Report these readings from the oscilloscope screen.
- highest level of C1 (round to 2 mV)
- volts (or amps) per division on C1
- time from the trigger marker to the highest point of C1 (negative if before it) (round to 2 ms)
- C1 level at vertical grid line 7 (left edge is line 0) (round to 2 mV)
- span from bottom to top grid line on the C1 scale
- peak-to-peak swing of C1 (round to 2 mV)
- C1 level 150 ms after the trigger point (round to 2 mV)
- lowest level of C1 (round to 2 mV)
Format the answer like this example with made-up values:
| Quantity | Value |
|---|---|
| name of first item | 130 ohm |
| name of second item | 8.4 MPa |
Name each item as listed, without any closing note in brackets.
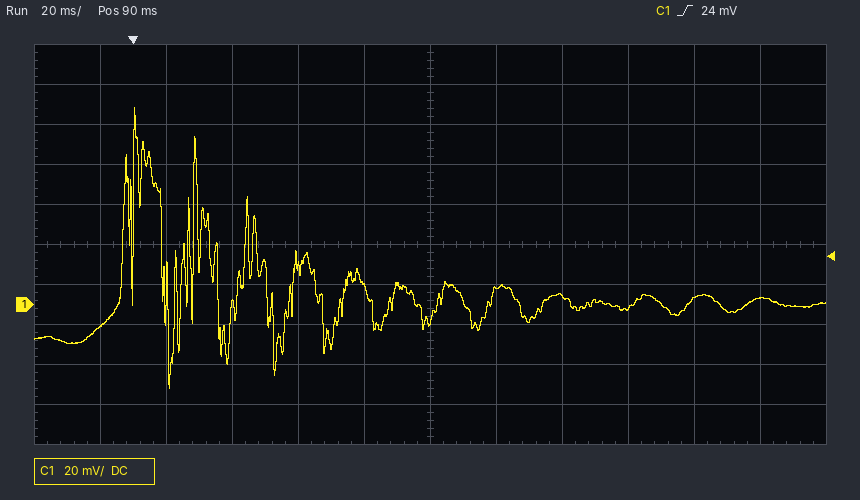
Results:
| Quantity | Value |
|---|---|
| highest level of C1 | 98 mV |
| volts (or amps) per division on C1 | 20 mV |
| time from the trigger marker to the highest point of C1 (negative if before it) | 0 ms |
| C1 level at vertical grid line 7 (left edge is line 0) | 8 mV |
| span from bottom to top grid line on the C1 scale | 200 mV |
| peak-to-peak swing of C1 | 140 mV |
| C1 level 150 ms after the trigger point | -2 mV |
| lowest level of C1 | -42 mV |
